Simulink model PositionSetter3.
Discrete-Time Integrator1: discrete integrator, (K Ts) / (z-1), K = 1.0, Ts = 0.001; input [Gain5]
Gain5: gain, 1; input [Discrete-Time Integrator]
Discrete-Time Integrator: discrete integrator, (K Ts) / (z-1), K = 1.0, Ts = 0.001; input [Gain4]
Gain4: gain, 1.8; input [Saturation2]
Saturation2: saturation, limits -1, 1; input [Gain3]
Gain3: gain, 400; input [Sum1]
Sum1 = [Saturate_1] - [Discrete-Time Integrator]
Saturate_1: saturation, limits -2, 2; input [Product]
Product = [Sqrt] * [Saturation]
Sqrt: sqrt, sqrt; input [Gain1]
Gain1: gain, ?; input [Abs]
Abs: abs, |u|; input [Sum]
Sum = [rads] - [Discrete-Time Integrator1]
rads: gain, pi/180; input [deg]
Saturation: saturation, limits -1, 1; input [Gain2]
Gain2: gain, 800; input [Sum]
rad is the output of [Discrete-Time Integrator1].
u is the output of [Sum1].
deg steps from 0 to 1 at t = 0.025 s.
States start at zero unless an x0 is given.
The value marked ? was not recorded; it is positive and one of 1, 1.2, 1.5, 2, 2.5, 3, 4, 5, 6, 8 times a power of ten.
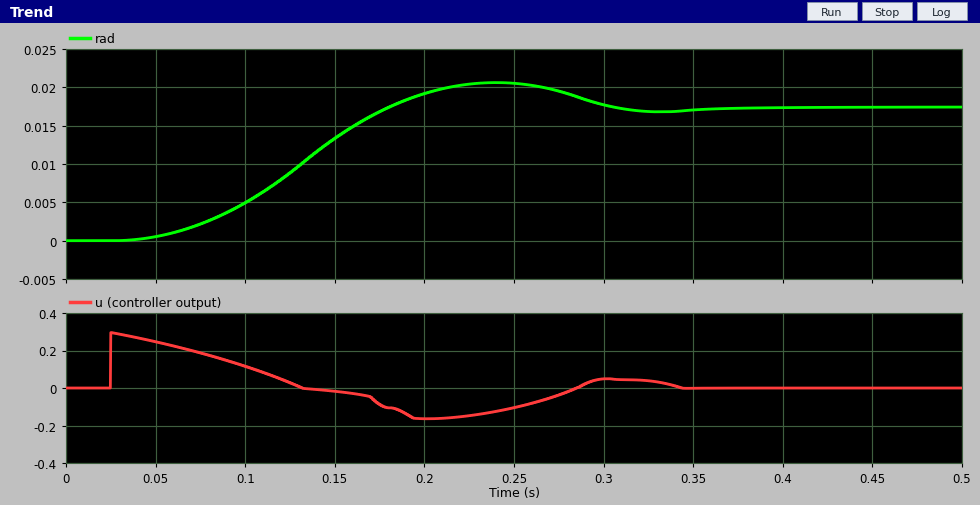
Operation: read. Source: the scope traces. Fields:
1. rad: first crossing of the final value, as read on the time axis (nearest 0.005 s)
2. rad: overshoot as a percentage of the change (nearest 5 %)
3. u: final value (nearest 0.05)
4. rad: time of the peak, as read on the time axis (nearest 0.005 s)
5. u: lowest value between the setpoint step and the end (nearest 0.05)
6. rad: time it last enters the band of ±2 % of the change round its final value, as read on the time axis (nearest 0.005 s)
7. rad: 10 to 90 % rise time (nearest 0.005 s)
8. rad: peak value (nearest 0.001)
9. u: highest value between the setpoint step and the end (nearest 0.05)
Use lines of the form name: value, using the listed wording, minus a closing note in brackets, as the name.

rad: first crossing of the final value, as read on the time axis: 0.180 s
rad: overshoot as a percentage of the change: 20 %
u: final value: 0.00
rad: time of the peak, as read on the time axis: 0.240 s
u: lowest value between the setpoint step and the end: -0.15
rad: time it last enters the band of ±2 % of the change round its final value, as read on the time axis: 0.355 s
rad: 10 to 90 % rise time: 0.095 s
rad: peak value: 0.021
u: highest value between the setpoint step and the end: 0.30
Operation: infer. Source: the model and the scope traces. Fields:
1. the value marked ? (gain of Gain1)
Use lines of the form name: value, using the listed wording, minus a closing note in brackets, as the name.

the value marked ?: 5
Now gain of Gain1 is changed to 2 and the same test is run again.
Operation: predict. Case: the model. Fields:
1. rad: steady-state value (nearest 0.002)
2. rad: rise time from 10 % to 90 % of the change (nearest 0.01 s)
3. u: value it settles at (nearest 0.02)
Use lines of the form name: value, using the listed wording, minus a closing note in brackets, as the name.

rad: steady-state value: 0.018
rad: rise time from 10 % to 90 % of the change: 0.13 s
u: value it settles at: 0.00
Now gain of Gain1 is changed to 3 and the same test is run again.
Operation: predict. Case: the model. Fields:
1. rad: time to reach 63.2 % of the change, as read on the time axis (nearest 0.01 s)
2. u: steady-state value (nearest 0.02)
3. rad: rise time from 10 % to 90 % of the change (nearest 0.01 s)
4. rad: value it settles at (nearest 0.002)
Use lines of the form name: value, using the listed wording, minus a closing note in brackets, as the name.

rad: time to reach 63.2 % of the change, as read on the time axis: 0.14 s
u: steady-state value: 0.00
rad: rise time from 10 % to 90 % of the change: 0.11 s
rad: value it settles at: 0.018
